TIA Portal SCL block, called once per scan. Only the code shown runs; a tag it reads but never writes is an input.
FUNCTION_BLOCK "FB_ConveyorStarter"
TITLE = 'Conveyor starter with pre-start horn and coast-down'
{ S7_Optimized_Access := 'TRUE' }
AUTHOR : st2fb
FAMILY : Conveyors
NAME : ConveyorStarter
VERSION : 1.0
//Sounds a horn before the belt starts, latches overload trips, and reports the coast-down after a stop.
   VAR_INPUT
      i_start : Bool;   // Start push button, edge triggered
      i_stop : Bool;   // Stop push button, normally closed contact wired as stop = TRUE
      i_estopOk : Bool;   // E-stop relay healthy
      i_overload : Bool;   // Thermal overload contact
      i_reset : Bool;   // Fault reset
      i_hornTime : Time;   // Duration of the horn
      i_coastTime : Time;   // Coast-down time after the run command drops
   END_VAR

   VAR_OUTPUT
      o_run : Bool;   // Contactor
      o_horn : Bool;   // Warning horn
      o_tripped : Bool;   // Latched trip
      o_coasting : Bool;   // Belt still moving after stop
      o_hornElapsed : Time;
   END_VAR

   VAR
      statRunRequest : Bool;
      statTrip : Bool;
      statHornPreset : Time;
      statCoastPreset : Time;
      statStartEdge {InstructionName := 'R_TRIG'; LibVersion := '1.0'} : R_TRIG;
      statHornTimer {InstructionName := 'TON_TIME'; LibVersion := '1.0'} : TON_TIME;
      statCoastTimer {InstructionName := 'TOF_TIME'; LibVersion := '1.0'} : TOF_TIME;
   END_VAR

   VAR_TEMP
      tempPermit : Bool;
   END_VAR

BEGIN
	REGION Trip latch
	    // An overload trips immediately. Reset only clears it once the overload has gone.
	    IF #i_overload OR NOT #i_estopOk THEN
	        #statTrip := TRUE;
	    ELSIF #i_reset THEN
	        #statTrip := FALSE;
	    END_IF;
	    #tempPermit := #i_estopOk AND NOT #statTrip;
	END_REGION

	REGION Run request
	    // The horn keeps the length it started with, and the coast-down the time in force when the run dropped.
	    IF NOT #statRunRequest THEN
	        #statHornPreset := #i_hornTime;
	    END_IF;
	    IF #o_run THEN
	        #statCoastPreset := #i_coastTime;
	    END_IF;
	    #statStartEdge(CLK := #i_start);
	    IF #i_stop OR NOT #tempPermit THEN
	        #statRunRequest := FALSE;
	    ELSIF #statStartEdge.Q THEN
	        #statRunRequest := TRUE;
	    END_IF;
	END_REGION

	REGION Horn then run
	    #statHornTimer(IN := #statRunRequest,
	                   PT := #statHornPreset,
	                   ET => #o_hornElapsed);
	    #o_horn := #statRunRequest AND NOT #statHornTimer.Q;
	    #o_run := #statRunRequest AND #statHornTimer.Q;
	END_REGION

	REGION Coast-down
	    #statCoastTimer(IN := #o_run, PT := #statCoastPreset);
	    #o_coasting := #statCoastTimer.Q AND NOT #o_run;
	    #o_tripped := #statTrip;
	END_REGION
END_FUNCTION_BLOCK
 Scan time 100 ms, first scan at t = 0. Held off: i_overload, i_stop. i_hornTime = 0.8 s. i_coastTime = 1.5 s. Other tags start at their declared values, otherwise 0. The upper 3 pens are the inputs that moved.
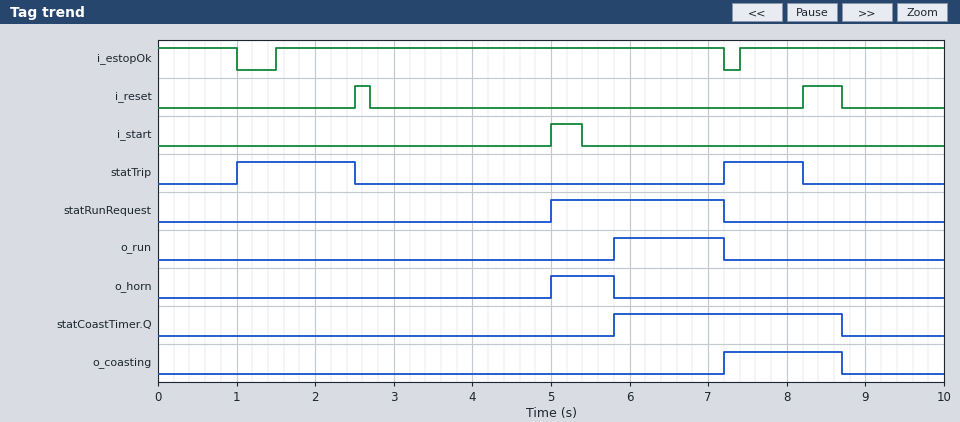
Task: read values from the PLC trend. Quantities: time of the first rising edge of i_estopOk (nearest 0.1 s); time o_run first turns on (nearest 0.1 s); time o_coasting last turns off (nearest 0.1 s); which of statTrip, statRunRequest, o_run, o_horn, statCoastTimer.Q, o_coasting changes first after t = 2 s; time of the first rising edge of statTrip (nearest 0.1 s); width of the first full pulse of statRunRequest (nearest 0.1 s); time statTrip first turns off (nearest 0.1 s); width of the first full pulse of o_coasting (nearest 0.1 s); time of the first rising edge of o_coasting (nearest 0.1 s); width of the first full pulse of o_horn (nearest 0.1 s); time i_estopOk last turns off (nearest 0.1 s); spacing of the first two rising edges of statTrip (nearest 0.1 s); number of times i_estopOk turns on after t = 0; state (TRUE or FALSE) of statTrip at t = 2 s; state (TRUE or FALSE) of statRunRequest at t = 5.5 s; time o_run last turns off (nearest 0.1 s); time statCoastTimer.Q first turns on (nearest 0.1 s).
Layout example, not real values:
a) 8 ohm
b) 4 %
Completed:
a) 1.5 s
b) 5.8 s
c) 8.7 s
d) statTrip
e) 1.0 s
f) 2.2 s
g) 2.5 s
h) 1.5 s
i) 7.2 s
j) 0.8 s
k) 7.2 s
l) 6.2 s
m) 2
n) TRUE
o) TRUE
p) 7.2 s
q) 5.8 s
